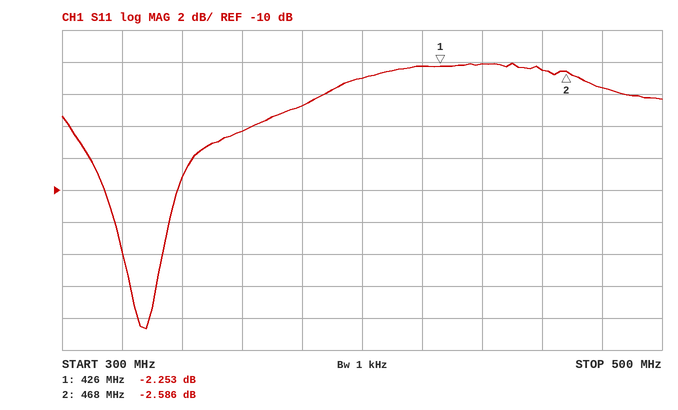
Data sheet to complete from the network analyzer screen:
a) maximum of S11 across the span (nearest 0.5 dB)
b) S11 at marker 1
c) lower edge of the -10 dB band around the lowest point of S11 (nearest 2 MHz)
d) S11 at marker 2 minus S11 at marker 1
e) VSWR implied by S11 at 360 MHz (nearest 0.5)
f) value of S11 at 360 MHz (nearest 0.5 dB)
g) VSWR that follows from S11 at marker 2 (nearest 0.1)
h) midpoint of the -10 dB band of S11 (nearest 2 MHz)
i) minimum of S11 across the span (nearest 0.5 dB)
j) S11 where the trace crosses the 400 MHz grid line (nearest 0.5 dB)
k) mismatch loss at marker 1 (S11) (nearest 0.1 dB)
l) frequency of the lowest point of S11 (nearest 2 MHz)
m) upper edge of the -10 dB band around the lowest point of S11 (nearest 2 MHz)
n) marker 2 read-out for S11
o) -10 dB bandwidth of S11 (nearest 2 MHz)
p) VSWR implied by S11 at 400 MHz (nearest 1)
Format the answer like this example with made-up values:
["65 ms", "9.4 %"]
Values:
["-2.0 dB", "-2.253 dB", "314 MHz", "-0.333 dB", "3.0", "-6.5 dB", "6.8", "326 MHz", "-18.5 dB", "-3.0 dB", "3.9 dB", "328 MHz", "338 MHz", "-2.586 dB", "24 MHz", "6"]
